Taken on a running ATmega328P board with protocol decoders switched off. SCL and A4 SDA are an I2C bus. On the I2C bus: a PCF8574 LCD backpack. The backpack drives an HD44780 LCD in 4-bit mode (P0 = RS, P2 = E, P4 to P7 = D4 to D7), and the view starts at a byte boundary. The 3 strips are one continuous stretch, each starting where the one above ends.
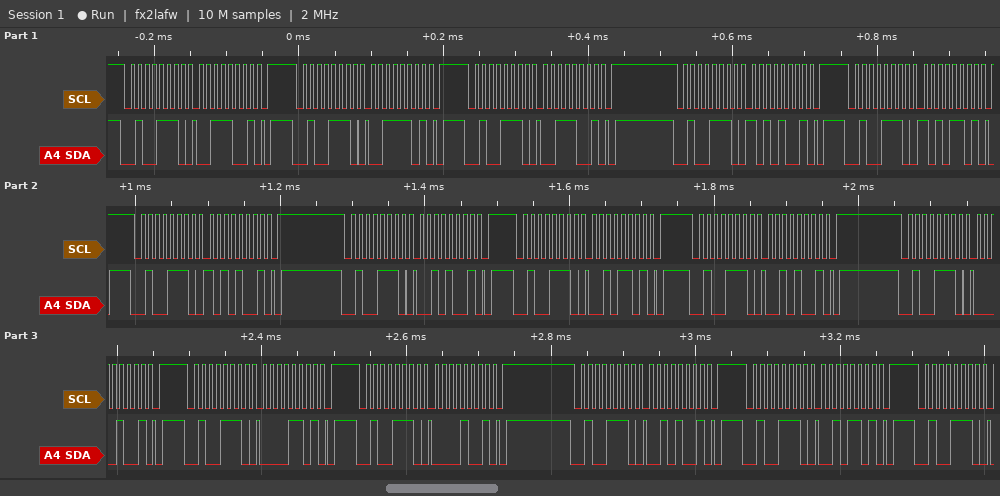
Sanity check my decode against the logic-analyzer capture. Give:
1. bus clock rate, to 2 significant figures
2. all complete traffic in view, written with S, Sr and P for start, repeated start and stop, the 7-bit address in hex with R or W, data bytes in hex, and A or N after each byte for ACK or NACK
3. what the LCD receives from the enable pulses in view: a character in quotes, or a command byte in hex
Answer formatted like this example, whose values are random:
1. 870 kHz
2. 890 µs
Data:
1. 100 kHz
2. S 27W A 39 A P S 27W A 3D A P S 27W A 39 A P S 27W A A9 A P S 27W A AD A P S 27W A A9 A P S 27W A 29 A P S 27W A 2D A P S 27W A 29 A P S 27W A 09 A P S 27W A 0D A P S 27W A 09 A P S 27W A 29 A P S 27W A 2D A P S 27W A
3. ':' ' '
